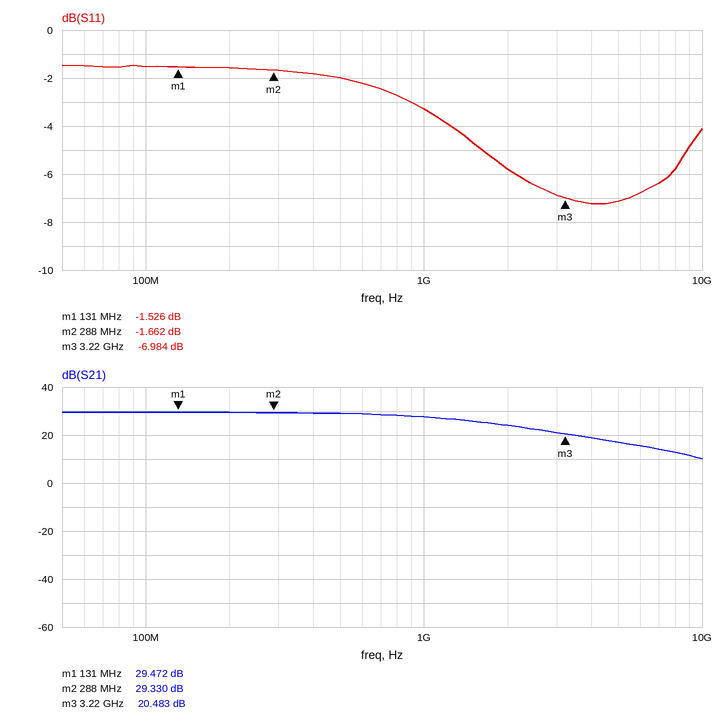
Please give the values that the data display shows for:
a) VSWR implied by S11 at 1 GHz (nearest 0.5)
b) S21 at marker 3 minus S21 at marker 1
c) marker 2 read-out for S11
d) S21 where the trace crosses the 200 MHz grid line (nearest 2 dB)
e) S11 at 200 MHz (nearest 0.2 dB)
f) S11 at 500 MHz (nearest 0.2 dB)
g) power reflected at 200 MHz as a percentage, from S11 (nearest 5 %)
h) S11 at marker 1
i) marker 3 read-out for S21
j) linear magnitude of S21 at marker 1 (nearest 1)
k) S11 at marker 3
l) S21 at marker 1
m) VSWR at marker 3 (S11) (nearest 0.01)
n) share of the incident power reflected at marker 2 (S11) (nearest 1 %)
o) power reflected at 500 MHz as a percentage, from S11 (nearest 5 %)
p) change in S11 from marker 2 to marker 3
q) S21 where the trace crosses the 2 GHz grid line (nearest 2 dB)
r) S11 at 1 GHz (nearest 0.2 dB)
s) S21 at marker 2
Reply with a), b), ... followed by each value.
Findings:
a) 5.5
b) -8.989 dB
c) -1.662 dB
d) 30 dB
e) -1.6 dB
f) -2.0 dB
g) 70 %
h) -1.526 dB
i) 20.483 dB
j) 30
k) -6.984 dB
l) 29.472 dB
m) 2.62
n) 68 %
o) 65 %
p) -5.322 dB
q) 24 dB
r) -3.2 dB
s) 29.330 dB
